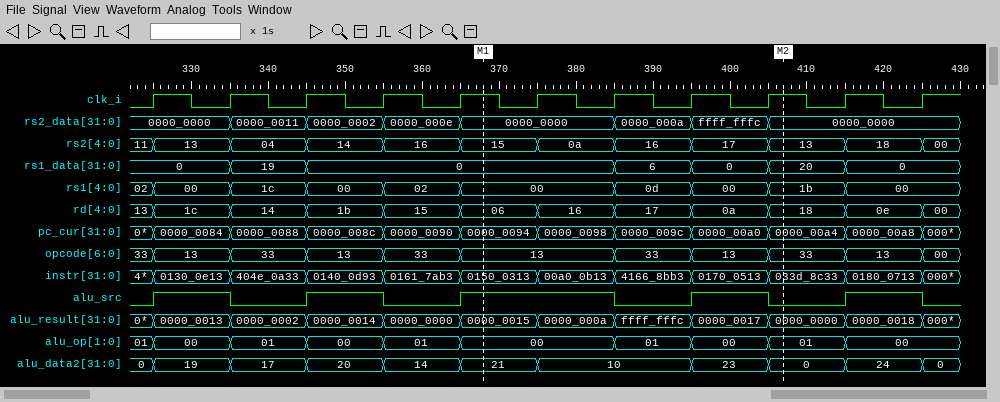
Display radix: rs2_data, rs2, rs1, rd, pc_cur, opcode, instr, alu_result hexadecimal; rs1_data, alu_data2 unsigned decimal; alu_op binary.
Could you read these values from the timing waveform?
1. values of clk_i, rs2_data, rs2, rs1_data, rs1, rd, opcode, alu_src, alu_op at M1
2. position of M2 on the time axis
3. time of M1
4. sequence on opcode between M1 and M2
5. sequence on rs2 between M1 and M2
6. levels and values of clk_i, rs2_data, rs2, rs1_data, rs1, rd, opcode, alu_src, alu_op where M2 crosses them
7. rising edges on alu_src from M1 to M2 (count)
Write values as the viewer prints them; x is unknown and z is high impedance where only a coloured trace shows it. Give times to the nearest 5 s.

clk_i=1, rs2_data=0000_0000, rs2=15, rs1_data=0, rs1=00, rd=06, opcode=13, alu_src=1, alu_op=00
405 s
370 s
13, 33, 13, 33
15, 0a, 16, 17, 13
clk_i=1, rs2_data=0000_0000, rs2=13, rs1_data=20, rs1=1b, rd=18, opcode=33, alu_src=0, alu_op=01
1
